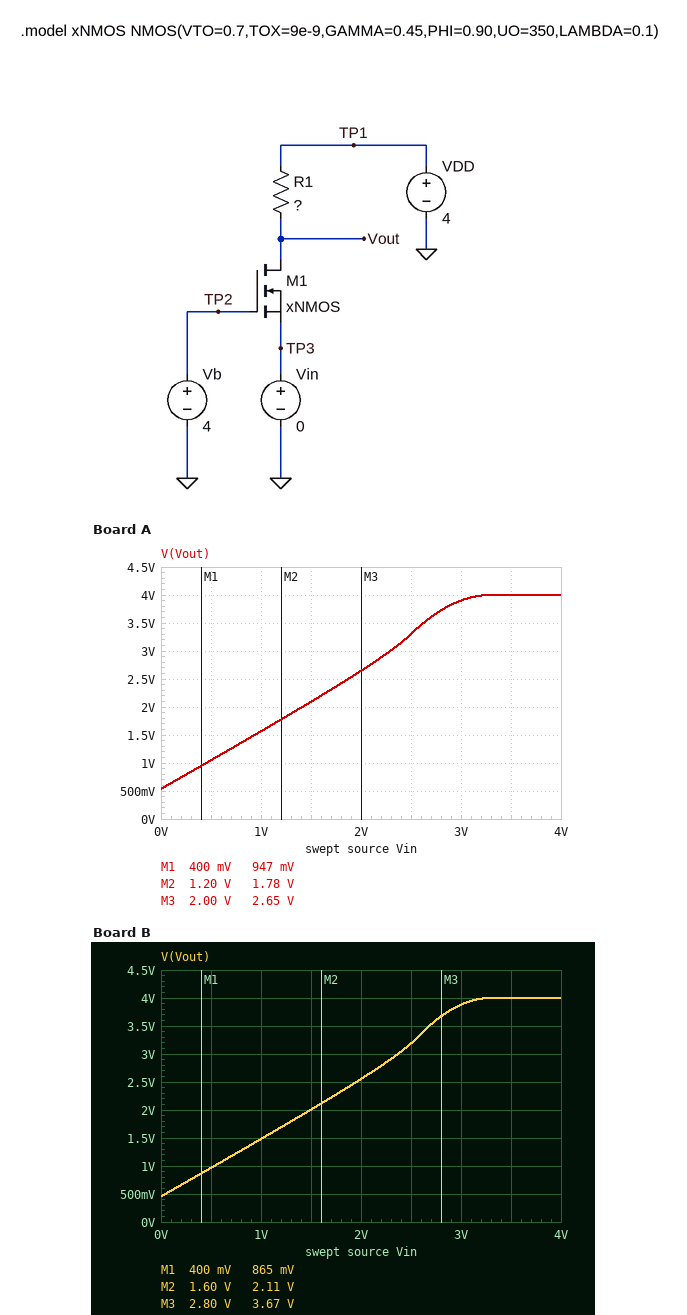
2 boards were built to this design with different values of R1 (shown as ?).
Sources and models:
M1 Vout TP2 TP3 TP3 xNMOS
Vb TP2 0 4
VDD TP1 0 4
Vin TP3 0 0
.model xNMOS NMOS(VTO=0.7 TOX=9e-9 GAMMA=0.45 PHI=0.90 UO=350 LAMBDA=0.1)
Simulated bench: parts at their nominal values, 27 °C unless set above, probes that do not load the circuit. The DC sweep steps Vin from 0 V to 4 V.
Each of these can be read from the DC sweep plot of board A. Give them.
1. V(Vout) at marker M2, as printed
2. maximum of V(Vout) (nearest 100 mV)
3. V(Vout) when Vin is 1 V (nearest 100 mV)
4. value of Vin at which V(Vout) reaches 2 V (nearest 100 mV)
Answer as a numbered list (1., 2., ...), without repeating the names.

1. 1.78 V
2. 4.0 V
3. 1.6 V
4. 1.4 V
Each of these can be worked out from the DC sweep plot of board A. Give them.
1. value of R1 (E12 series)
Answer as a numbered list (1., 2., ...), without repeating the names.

1. 15 kΩ
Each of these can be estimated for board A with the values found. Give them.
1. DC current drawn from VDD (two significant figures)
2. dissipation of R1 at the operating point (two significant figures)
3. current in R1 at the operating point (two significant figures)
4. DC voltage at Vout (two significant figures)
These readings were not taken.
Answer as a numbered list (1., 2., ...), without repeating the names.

1. 230 µA
2. 800 µW
3. 230 µA
4. 540 mV
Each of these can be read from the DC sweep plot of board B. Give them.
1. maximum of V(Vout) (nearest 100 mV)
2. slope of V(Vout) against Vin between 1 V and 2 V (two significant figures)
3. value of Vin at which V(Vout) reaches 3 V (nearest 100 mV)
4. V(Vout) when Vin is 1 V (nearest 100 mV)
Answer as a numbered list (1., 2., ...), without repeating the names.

1. 4.0 V
2. 1.1 V/V
3. 2.4 V
4. 1.5 V
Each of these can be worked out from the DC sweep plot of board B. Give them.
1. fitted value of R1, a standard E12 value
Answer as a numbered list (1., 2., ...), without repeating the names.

1. 18 kΩ
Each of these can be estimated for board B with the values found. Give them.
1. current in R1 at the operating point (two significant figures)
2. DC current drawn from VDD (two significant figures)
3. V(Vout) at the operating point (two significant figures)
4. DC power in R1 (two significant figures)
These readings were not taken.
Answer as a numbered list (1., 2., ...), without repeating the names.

1. 200 µA
2. 200 µA
3. 460 mV
4. 700 µW
